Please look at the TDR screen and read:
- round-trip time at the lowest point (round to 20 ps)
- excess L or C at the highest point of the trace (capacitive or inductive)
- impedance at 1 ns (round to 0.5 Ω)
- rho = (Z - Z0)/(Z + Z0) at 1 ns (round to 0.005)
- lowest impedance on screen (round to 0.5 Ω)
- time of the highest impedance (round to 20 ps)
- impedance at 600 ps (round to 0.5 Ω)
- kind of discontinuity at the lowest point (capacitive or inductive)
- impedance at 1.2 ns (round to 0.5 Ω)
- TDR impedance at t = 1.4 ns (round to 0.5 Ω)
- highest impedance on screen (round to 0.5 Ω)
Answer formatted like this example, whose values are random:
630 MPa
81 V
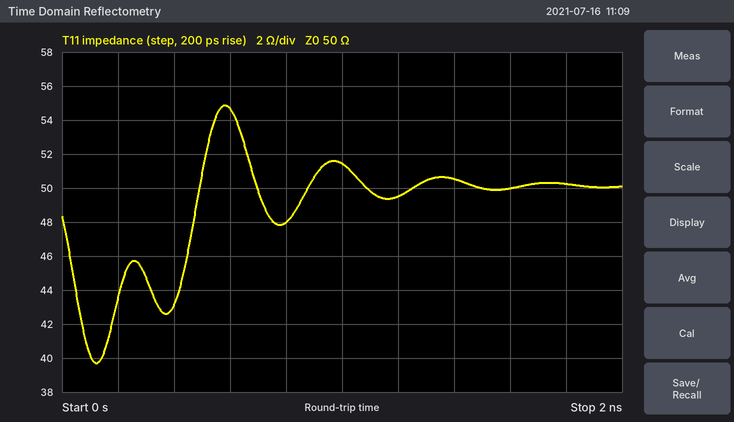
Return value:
120 ps
inductive
51.5 Ω
+0.015
39.5 Ω
580 ps
54.5 Ω
capacitive
49.5 Ω
50.5 Ω
55.0 Ω
